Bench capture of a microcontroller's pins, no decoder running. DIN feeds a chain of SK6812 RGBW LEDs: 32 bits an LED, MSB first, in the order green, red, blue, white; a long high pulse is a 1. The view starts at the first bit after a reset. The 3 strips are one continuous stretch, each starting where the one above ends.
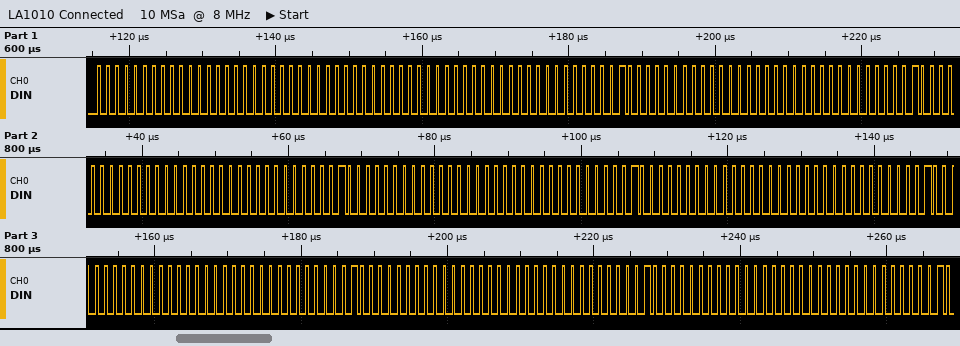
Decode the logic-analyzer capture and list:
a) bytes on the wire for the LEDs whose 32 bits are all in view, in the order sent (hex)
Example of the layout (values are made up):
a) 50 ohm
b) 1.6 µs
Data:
a) 00 00 00 00 00 00 00 40 00 00 00 40 00 00 00 40 00 00 00 40 00 00 00 40 00 00 00 40 00 00 00 40
